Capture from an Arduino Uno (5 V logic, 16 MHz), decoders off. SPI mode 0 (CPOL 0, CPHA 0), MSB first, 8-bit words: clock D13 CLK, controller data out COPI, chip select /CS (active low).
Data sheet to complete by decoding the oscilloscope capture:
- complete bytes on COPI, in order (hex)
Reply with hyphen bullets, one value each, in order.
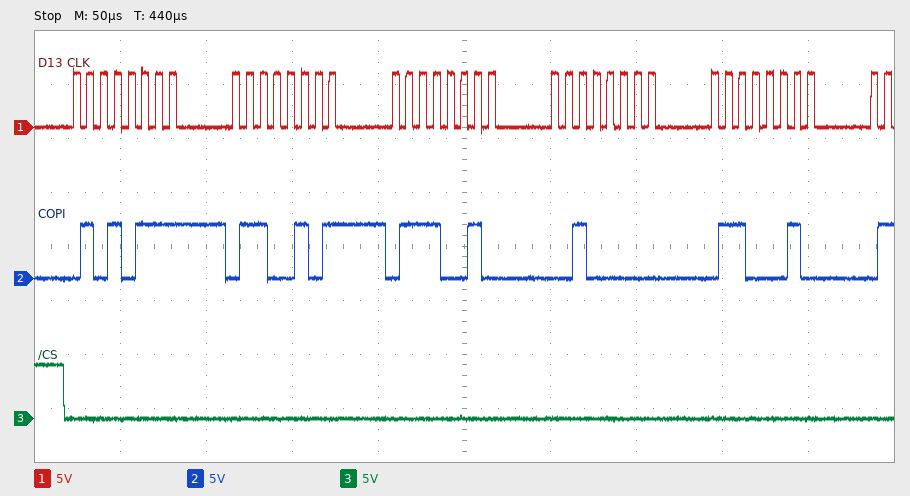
- 0x57 0x65 0x72 0x20 0x62
